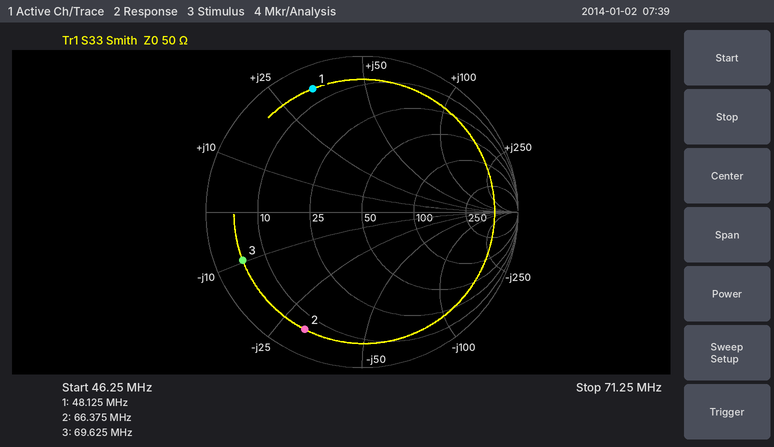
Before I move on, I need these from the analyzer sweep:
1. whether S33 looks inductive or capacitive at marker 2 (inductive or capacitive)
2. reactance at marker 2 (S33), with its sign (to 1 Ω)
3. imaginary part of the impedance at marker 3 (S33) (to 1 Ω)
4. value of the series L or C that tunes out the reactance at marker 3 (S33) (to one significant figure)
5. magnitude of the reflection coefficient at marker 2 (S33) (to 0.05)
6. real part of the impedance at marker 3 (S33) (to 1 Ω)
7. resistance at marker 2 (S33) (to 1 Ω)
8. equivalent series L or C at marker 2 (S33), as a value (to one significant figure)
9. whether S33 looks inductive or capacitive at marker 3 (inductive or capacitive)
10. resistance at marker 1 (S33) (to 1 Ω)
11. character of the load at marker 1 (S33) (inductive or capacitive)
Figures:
capacitive
-31 Ω
-10 Ω
20 nH
0.85
5 Ω
6 Ω
80 pF
capacitive
6 Ω
inductive
